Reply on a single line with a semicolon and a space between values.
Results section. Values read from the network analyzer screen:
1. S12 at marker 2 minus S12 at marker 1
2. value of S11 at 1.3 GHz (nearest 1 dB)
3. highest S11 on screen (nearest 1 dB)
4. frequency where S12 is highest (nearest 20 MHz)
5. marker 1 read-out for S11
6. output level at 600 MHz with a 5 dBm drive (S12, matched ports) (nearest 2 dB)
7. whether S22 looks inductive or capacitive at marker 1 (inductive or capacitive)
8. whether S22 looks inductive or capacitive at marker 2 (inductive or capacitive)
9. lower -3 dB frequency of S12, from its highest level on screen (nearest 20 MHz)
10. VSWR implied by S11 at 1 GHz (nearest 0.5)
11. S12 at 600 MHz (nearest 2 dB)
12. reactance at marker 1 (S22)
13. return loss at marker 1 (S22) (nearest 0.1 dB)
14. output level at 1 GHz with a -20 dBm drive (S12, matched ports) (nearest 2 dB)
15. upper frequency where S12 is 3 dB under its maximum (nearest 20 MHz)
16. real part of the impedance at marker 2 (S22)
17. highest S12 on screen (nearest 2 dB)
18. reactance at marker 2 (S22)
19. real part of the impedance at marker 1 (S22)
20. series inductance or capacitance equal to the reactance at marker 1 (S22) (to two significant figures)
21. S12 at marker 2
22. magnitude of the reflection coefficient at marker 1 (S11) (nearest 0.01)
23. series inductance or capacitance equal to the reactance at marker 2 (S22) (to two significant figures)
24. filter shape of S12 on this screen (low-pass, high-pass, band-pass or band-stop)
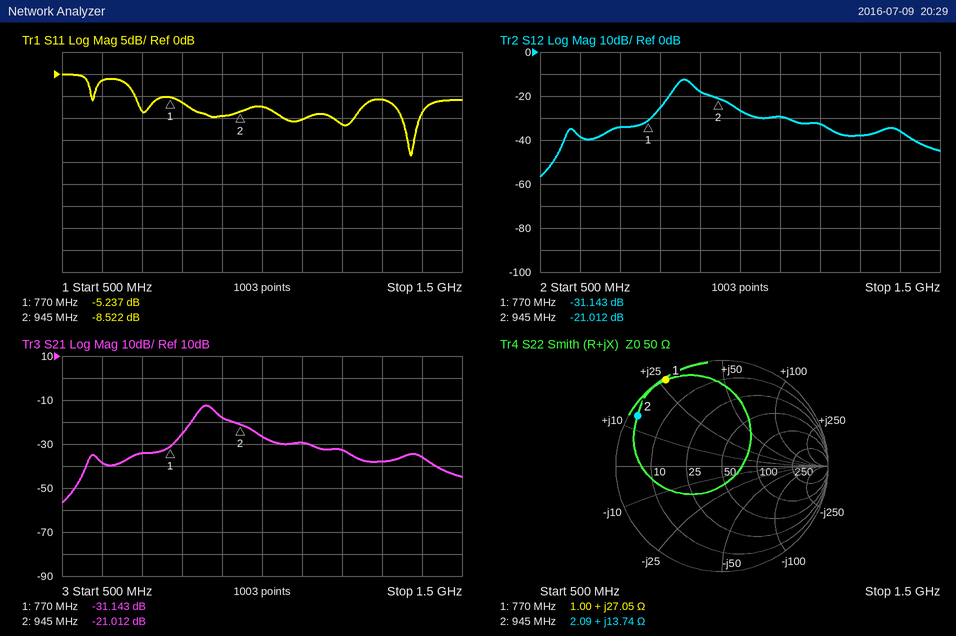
10.131 dB; -6 dB; 0 dB; 860 MHz; -5.237 dB; -34 dBm; inductive; inductive; 840 MHz; 2.5; -38 dB; +27.05 Ω; 0.3 dB; -46 dBm; 880 MHz; 2.09 Ω; -12 dB; +13.74 Ω; 1.00 Ω; 5.6 nH; -21.012 dB; 0.55; 2.3 nH; band-pass
